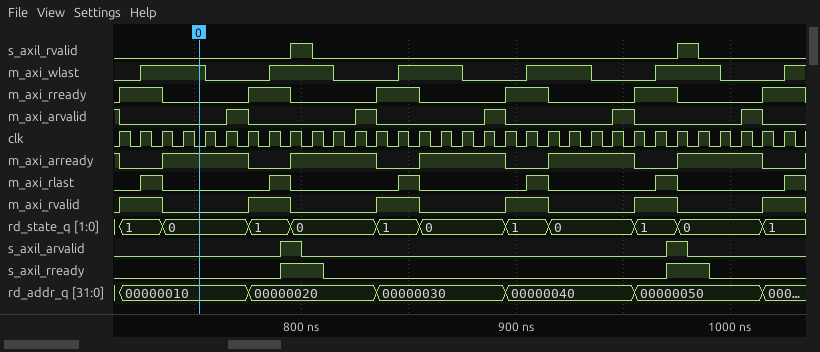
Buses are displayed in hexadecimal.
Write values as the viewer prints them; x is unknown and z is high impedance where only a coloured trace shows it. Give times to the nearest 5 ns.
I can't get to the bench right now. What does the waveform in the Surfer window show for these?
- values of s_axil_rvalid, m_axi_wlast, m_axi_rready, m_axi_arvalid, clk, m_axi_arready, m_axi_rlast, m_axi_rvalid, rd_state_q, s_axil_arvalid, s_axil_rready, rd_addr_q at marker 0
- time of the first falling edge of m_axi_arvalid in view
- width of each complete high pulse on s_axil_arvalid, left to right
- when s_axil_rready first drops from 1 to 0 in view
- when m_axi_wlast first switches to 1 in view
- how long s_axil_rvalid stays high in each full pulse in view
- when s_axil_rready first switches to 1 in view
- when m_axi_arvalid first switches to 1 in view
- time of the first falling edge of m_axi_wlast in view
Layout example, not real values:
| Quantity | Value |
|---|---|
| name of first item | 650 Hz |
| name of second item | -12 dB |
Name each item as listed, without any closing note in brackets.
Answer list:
| Quantity | Value |
|---|---|
| values of s_axil_rvalid, m_axi_wlast, m_axi_rready, m_axi_arvalid, clk, m_axi_arready, m_axi_rlast, m_axi_rvalid, rd_state_q, s_axil_arvalid, s_axil_rready, rd_addr_q at marker 0 | s_axil_rvalid=0, m_axi_wlast=1, m_axi_rready=0, m_axi_arvalid=0, clk=0, m_axi_arready=1, m_axi_rlast=0, m_axi_rvalid=0, rd_state_q=0, s_axil_arvalid=0, s_axil_rready=0, rd_addr_q=00000010 |
| time of the first falling edge of m_axi_arvalid in view | 715 ns |
| width of each complete high pulse on s_axil_arvalid, left to right | 10 ns, 10 ns |
| when s_axil_rready first drops from 1 to 0 in view | 810 ns |
| when m_axi_wlast first switches to 1 in view | 725 ns |
| how long s_axil_rvalid stays high in each full pulse in view | 10 ns, 10 ns |
| when s_axil_rready first switches to 1 in view | 790 ns |
| when m_axi_arvalid first switches to 1 in view | 765 ns |
| time of the first falling edge of m_axi_wlast in view | 755 ns |
